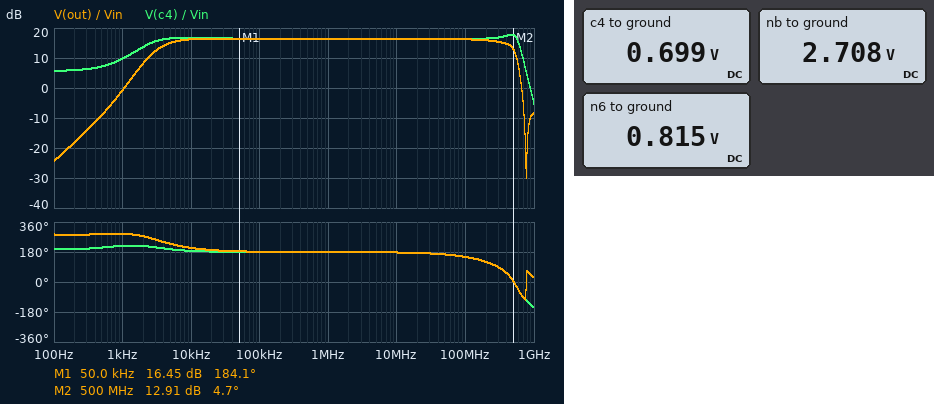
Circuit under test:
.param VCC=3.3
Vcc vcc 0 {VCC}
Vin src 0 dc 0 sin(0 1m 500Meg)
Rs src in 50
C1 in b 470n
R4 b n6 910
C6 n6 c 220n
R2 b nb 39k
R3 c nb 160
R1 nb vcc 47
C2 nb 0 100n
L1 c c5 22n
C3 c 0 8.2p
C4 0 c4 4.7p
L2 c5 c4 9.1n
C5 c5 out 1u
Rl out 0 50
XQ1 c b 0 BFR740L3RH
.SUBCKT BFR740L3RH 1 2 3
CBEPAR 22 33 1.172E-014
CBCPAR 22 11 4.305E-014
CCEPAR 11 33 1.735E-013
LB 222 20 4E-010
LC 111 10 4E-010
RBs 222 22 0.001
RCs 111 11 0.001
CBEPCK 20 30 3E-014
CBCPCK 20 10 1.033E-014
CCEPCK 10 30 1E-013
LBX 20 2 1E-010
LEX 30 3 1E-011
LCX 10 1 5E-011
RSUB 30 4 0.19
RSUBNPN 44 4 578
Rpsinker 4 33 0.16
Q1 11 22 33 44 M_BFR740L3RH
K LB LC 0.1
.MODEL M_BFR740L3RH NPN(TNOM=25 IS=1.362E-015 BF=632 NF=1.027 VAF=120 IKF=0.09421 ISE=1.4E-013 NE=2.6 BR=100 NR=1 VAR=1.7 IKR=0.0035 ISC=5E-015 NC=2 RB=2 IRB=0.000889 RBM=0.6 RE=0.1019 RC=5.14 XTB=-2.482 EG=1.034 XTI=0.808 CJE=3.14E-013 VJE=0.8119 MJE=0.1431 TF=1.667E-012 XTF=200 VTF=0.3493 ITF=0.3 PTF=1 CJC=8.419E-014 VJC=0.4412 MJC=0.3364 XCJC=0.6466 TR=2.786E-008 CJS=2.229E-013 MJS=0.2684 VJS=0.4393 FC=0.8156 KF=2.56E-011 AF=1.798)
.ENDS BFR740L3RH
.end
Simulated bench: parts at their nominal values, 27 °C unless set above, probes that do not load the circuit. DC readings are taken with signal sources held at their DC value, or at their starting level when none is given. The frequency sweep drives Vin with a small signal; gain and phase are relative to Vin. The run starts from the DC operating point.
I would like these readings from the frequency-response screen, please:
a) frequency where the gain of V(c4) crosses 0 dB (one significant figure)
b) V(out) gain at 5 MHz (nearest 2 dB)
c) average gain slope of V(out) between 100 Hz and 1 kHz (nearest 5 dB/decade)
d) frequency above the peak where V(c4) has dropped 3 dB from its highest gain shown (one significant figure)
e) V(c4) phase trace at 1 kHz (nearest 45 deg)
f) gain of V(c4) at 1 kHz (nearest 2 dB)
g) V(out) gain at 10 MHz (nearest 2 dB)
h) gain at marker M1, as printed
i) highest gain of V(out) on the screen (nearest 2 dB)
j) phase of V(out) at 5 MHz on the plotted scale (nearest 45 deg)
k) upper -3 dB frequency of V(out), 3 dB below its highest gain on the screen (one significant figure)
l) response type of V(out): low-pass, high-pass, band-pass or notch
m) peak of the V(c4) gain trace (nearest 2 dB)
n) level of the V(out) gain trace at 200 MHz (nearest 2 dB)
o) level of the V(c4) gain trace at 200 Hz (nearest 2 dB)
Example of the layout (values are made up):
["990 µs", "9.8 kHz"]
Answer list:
["900 MHz", "16 dB", "25 dB/decade", "600 MHz", "225 deg", "10 dB", "16 dB", "16.45 dB", "16 dB", "180 deg", "500 MHz", "band-pass", "18 dB", "16 dB", "6 dB"]
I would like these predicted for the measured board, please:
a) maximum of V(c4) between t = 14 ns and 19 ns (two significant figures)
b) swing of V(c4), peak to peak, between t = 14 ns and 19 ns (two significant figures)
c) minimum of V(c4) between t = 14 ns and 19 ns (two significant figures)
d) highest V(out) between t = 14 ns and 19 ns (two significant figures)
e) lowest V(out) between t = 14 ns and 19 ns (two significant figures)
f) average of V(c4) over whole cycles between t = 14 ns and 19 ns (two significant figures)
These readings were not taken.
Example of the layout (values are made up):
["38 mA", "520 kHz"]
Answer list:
["710 mV", "15 mV", "690 mV", "4.4 mV", "-4.4 mV", "700 mV"]
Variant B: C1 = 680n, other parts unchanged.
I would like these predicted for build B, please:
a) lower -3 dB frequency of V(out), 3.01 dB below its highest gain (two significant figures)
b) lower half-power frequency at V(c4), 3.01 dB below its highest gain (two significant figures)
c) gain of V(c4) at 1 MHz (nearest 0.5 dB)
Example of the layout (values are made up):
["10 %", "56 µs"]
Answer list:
["2.9 kHz", "1.5 kHz", "16.5 dB"]
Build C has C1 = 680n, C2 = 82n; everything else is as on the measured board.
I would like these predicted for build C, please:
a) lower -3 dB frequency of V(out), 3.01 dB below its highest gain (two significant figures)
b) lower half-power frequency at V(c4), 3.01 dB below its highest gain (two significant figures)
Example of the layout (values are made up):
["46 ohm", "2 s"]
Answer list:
["2.9 kHz", "1.5 kHz"]
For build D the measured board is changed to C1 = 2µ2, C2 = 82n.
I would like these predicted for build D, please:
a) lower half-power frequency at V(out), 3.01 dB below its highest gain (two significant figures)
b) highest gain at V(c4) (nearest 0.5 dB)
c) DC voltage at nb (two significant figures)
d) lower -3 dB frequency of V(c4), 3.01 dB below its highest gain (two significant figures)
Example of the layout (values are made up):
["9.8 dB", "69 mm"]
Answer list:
["1.8 kHz", "20.0 dB", "2.7 V", "30 Hz"]
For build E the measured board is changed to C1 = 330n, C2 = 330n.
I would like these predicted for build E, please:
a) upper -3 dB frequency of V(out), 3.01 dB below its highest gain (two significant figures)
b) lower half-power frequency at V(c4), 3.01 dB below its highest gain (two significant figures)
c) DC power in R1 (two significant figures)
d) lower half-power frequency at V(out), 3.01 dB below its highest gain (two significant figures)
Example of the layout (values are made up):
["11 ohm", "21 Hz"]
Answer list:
["490 MHz", "4.0 kHz", "7.5 mW", "4.5 kHz"]
